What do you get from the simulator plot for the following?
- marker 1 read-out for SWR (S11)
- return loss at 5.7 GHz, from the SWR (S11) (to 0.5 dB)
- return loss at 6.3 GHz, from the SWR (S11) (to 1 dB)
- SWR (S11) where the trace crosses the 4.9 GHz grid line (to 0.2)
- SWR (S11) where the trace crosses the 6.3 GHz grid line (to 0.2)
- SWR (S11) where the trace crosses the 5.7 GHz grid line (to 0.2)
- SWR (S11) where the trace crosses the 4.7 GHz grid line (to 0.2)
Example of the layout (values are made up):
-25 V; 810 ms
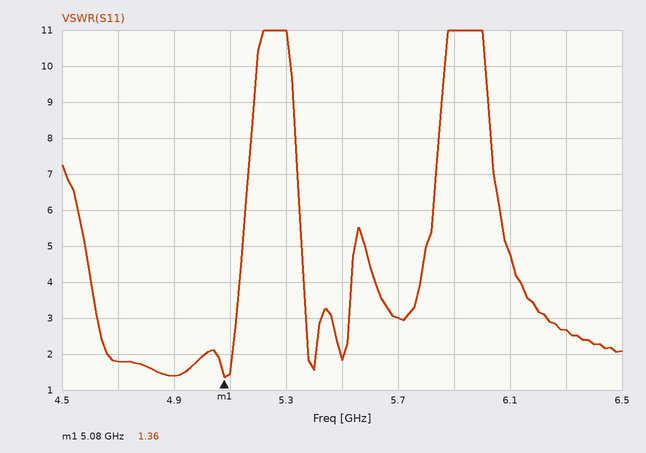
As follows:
1.36; 6.0 dB; 7 dB; 1.4; 2.6; 3.0; 1.8
